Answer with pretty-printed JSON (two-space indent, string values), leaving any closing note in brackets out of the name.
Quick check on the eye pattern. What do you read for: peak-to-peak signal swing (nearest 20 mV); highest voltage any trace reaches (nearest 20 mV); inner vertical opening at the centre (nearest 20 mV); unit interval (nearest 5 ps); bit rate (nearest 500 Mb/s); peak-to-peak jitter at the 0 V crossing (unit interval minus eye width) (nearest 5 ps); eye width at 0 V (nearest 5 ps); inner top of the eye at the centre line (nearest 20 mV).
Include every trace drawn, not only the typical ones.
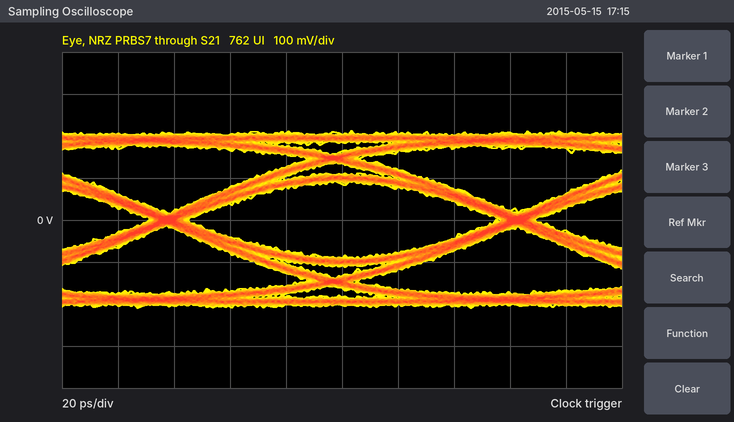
{
  "peak-to-peak signal swing": "420 mV",
  "highest voltage any trace reaches": "220 mV",
  "inner vertical opening at the centre": "180 mV",
  "unit interval": "125 ps",
  "bit rate": "8.0 Gb/s",
  "peak-to-peak jitter at the 0 V crossing (unit interval minus eye width)": "15 ps",
  "eye width at 0 V": "110 ps",
  "inner top of the eye at the centre line": "80 mV"
}
